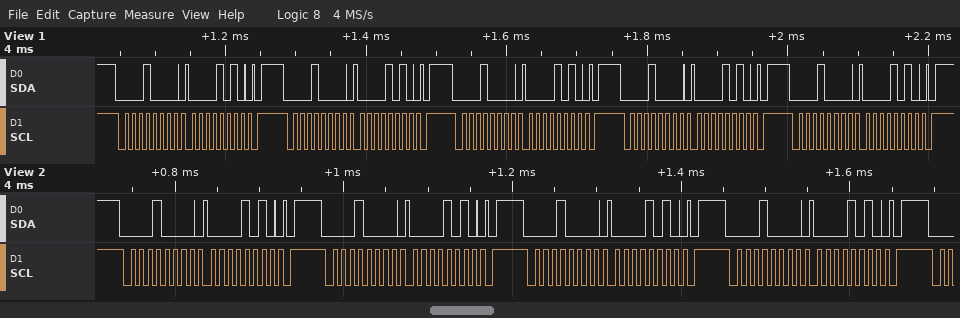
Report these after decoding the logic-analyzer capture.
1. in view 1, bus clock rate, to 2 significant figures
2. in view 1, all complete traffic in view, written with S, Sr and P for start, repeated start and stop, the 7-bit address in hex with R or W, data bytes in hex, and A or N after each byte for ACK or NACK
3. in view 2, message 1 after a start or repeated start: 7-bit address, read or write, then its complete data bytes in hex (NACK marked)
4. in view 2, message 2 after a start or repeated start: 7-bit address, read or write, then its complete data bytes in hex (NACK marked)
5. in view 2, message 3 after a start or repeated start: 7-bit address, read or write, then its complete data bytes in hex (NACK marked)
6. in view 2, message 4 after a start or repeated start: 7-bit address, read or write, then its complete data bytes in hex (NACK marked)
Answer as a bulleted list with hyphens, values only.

- 100 kHz
- S 08W A 0A A P S 08W A 0A A P S 08W A 0A A P S 08W A 0A A P S 08W A 0A A P
- 0x08 write: 0A
- 0x08 write: 0A
- 0x08 write: 0A
- 0x08 write: 0A
